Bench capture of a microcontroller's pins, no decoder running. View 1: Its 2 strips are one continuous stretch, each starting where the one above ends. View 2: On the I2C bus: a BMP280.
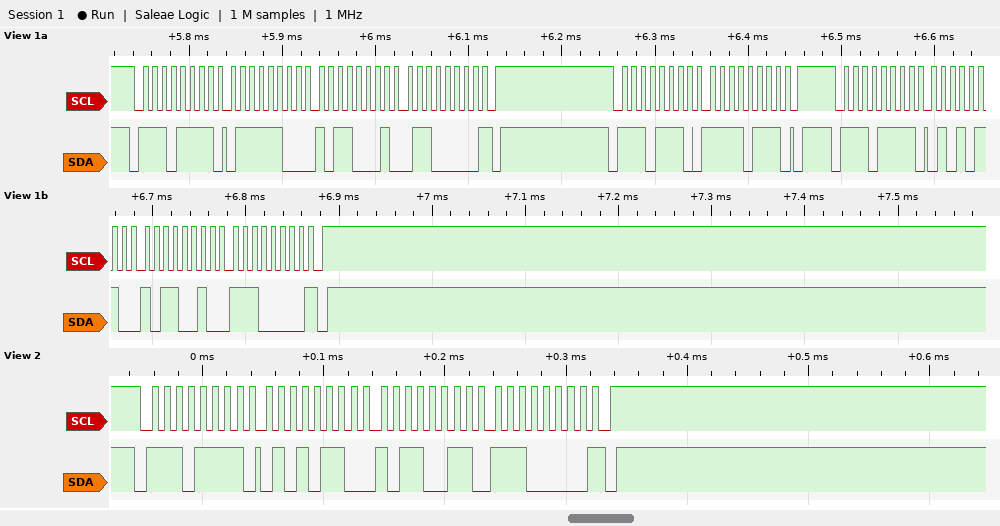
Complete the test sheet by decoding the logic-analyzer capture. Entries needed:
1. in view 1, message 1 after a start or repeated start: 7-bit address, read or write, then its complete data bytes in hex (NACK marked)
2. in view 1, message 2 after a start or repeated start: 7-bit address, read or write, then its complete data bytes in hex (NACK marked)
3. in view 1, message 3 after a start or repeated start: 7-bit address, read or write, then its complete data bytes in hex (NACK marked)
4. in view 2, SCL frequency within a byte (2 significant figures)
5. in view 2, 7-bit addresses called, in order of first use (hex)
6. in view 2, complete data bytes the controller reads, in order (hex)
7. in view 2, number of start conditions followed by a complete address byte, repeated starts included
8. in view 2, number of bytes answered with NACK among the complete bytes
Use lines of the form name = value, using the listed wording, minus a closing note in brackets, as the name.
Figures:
in view 1, message 1 after a start or repeated start: 7-bit address, read or write, then its complete data bytes in hex = 0x77 read: 7C B1 60 NACK
in view 1, message 2 after a start or repeated start: 7-bit address, read or write, then its complete data bytes in hex = 0x77 write: F7
in view 1, message 3 after a start or repeated start: 7-bit address, read or write, then its complete data bytes in hex = 0x77 read: 56 B2 E0 NACK
in view 2, SCL frequency within a byte = 100 kHz
in view 2, 7-bit addresses called, in order of first use = 0x77
in view 2, complete data bytes the controller reads, in order = 56 B3 E0
in view 2, number of start conditions followed by a complete address byte, repeated starts included = 1
in view 2, number of bytes answered with NACK among the complete bytes = 1
